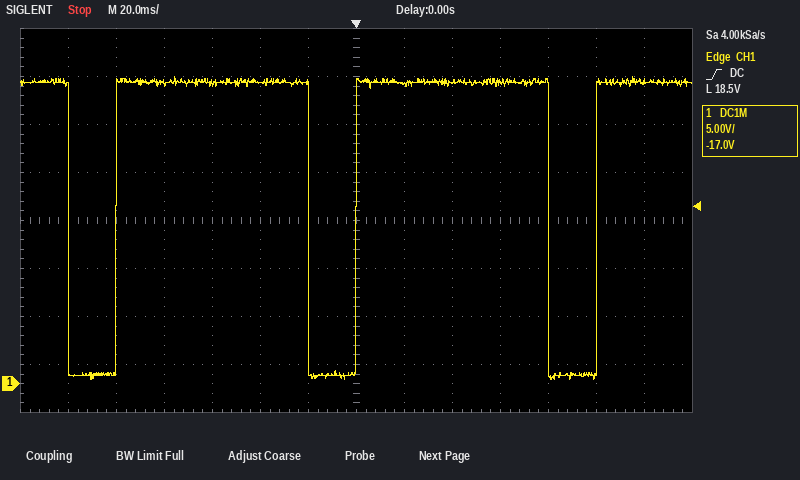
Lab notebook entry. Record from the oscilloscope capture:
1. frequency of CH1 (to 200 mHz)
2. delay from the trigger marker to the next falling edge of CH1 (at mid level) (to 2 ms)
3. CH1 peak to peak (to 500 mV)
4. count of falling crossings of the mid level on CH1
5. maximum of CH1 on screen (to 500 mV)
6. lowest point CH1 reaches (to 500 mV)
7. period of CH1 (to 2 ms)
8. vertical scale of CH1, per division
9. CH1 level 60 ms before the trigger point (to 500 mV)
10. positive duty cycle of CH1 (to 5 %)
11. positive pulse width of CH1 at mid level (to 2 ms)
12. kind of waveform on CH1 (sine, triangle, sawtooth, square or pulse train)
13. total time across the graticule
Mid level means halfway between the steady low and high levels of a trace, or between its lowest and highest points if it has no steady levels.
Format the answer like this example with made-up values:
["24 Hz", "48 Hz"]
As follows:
["10.0 Hz", "80 ms", "31.5 V", "3", "32.0 V", "500 mV", "100 ms", "5 V", "31.5 V", "80 %", "80 ms", "pulse train", "280 ms"]
